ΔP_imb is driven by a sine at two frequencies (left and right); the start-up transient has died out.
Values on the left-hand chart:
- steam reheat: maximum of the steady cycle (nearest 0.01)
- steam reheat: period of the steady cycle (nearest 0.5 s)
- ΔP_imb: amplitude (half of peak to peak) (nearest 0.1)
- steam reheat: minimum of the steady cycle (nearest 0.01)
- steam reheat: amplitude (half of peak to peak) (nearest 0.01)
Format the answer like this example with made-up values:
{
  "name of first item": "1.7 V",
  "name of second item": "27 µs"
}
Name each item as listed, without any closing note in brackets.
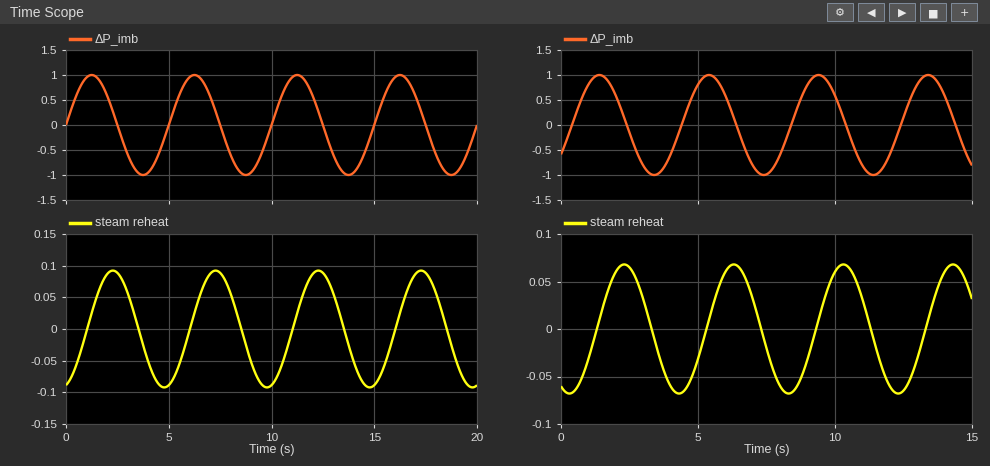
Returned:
{
  "steam reheat: maximum of the steady cycle": "0.09",
  "steam reheat: period of the steady cycle": "5.0 s",
  "ΔP_imb: amplitude (half of peak to peak)": "1.0",
  "steam reheat: minimum of the steady cycle": "-0.09",
  "steam reheat: amplitude (half of peak to peak)": "0.09"
}
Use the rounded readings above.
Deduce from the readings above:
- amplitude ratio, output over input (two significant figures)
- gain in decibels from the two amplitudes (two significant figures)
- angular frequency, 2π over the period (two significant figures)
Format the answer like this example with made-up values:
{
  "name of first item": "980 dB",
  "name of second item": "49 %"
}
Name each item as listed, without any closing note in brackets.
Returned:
{
  "amplitude ratio, output over input": "0.090",
  "gain in decibels from the two amplitudes": "-21 dB",
  "angular frequency, 2π over the period": "1.3 rad/s"
}
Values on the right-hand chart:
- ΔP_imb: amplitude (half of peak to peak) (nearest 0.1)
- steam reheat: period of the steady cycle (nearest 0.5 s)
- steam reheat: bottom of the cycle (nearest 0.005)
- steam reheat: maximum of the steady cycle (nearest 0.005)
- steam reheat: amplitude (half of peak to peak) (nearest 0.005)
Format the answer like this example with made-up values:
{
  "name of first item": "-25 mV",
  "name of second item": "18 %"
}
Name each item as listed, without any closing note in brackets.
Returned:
{
  "ΔP_imb: amplitude (half of peak to peak)": "1.0",
  "steam reheat: period of the steady cycle": "4.0 s",
  "steam reheat: bottom of the cycle": "-0.070",
  "steam reheat: maximum of the steady cycle": "0.070",
  "steam reheat: amplitude (half of peak to peak)": "0.070"
}
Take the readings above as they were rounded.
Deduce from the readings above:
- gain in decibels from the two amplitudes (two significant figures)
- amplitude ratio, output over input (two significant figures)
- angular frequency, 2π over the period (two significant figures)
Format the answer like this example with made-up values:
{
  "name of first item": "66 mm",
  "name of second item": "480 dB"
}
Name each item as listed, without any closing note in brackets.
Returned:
{
  "gain in decibels from the two amplitudes": "-23 dB",
  "amplitude ratio, output over input": "0.070",
  "angular frequency, 2π over the period": "1.6 rad/s"
}
